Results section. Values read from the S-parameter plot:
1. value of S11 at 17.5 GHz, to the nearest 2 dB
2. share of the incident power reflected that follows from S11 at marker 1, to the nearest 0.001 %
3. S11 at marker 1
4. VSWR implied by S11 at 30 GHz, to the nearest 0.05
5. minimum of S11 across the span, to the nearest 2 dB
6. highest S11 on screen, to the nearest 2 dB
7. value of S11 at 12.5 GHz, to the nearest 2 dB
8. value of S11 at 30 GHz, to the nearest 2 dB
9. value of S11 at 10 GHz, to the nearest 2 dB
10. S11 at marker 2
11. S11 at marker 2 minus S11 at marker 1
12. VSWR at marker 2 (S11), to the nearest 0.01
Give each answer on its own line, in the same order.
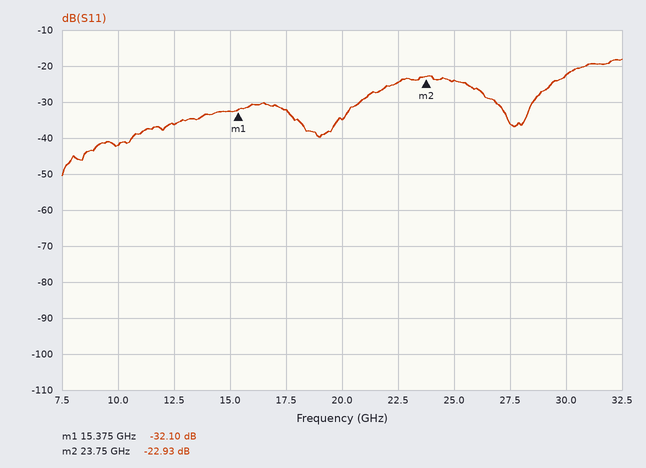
-32 dB
0.062 %
-32.10 dB
1.15
-50 dB
-18 dB
-36 dB
-22 dB
-42 dB
-22.93 dB
9.17 dB
1.15
